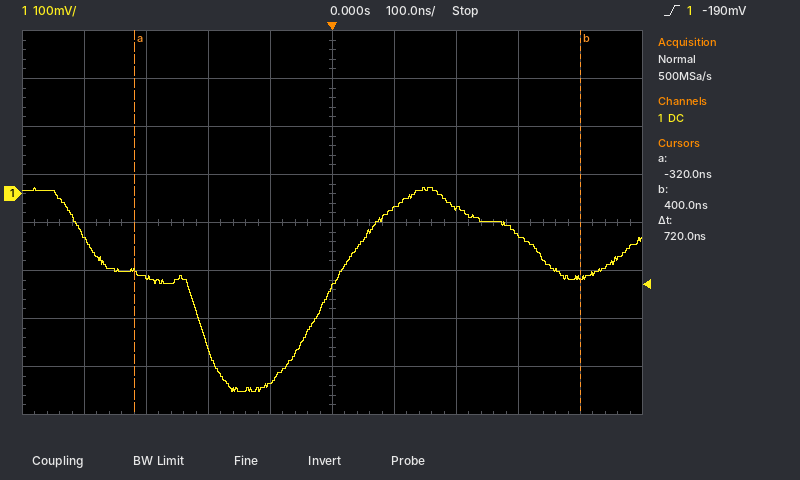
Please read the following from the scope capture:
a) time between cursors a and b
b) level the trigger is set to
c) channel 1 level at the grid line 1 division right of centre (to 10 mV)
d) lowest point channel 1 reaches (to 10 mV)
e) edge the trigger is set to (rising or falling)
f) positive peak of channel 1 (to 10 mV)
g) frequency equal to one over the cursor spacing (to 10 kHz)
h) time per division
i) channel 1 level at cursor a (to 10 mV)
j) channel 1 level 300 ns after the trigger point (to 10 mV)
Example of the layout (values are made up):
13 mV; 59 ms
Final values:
720 ns; -190 mV; -30 mV; -410 mV; rising; 10 mV; 1.39 MHz; 100 ns; -160 mV; -90 mV
